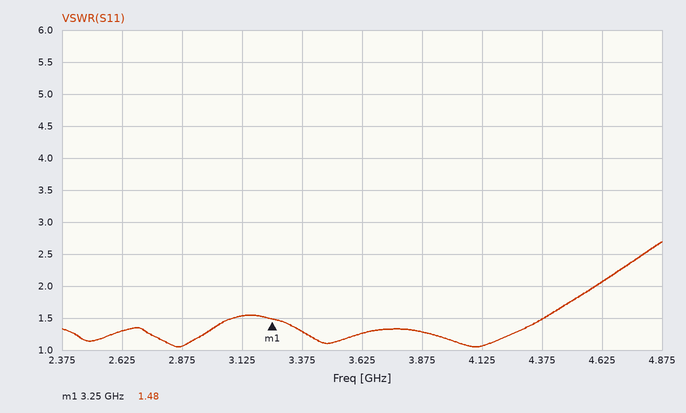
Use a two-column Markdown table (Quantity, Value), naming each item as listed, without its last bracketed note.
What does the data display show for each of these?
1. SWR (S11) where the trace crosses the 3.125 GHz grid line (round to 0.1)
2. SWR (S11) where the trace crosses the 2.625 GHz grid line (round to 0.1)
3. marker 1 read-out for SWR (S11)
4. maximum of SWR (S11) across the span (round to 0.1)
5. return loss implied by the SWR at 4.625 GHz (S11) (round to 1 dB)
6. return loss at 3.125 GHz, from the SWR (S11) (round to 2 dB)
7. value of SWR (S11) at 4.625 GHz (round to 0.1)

| Quantity | Value |
|---|---|
| SWR (S11) where the trace crosses the 3.125 GHz grid line | 1.5 |
| SWR (S11) where the trace crosses the 2.625 GHz grid line | 1.3 |
| marker 1 read-out for SWR | 1.48 |
| maximum of SWR (S11) across the span | 2.7 |
| return loss implied by the SWR at 4.625 GHz (S11) | 9 dB |
| return loss at 3.125 GHz, from the SWR (S11) | 14 dB |
| value of SWR (S11) at 4.625 GHz | 2.1 |
